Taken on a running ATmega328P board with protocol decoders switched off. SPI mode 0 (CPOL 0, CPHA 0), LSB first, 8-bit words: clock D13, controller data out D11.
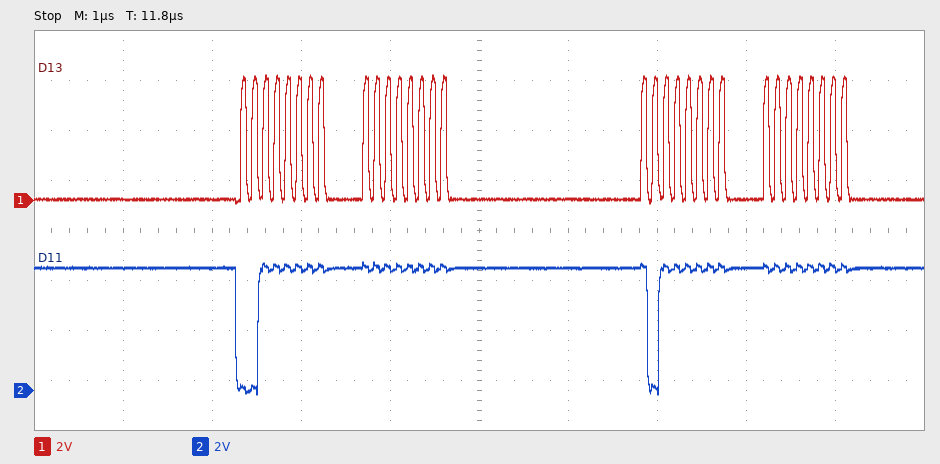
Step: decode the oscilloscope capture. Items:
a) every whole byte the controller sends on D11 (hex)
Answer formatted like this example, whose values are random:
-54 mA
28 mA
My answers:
FC FF FD FF
